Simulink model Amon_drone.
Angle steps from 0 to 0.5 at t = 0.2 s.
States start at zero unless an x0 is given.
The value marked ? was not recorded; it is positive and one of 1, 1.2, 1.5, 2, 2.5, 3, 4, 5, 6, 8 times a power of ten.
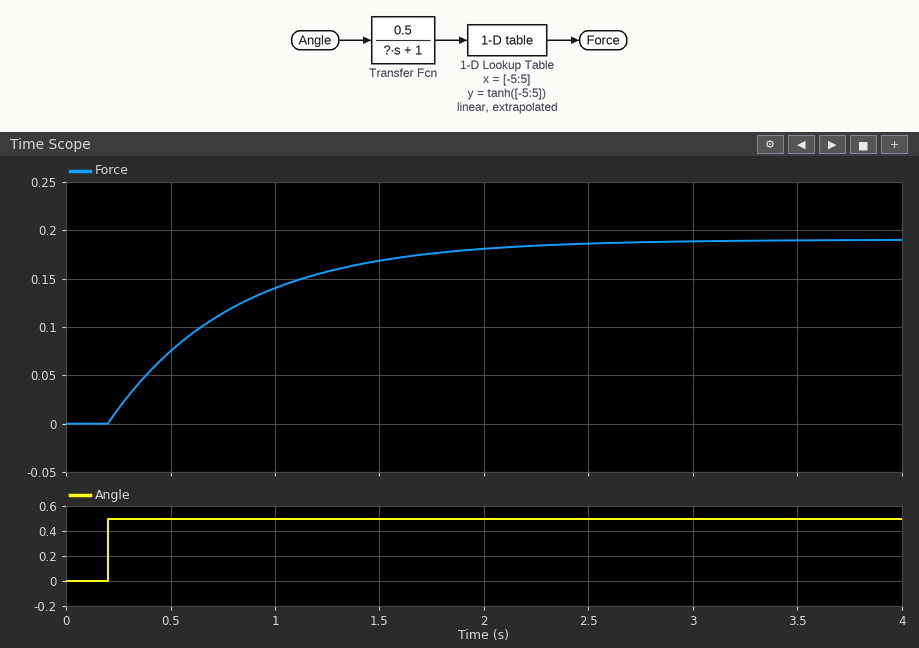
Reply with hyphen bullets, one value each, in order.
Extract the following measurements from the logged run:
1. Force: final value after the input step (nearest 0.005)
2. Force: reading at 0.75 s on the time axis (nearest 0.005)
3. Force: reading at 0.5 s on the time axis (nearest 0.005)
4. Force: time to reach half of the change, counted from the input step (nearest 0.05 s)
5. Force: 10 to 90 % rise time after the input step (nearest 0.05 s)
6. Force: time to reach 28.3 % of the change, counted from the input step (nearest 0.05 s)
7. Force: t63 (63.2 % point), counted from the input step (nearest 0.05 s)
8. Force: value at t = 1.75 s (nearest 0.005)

- 0.190
- 0.115
- 0.075
- 0.40 s
- 1.30 s
- 0.20 s
- 0.60 s
- 0.175
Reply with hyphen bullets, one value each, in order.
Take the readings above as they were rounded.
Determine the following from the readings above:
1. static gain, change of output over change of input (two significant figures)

- 0.38
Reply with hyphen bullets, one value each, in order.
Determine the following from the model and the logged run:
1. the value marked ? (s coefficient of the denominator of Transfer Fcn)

- 0.6
